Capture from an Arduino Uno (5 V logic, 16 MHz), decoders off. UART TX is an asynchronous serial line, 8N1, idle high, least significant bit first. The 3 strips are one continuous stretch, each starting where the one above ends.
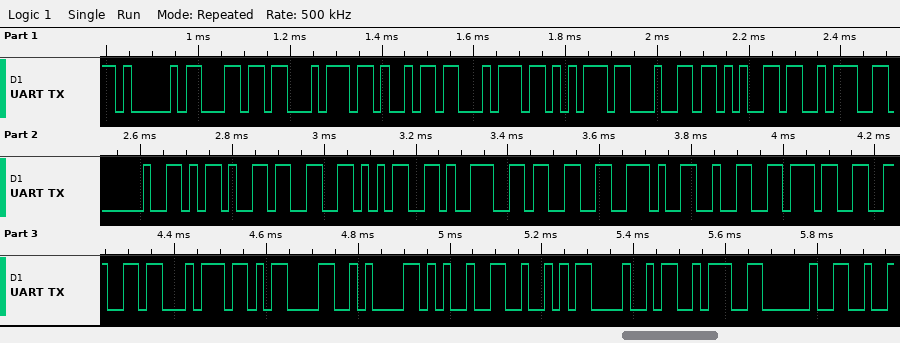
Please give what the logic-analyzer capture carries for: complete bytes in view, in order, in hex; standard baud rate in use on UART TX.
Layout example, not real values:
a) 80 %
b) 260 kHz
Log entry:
a) 0x41 0x6C 0x74 0x69 0x74 0x75 0x64 0x65 0x3A 0x20 0x2D 0x33 0x35 0x39 0x33 0x2E 0x32 0x37 0x66 0x74 0x0D 0x0A 0x25 0x52 0x48 0x3A 0x20
b) 57600 baud
